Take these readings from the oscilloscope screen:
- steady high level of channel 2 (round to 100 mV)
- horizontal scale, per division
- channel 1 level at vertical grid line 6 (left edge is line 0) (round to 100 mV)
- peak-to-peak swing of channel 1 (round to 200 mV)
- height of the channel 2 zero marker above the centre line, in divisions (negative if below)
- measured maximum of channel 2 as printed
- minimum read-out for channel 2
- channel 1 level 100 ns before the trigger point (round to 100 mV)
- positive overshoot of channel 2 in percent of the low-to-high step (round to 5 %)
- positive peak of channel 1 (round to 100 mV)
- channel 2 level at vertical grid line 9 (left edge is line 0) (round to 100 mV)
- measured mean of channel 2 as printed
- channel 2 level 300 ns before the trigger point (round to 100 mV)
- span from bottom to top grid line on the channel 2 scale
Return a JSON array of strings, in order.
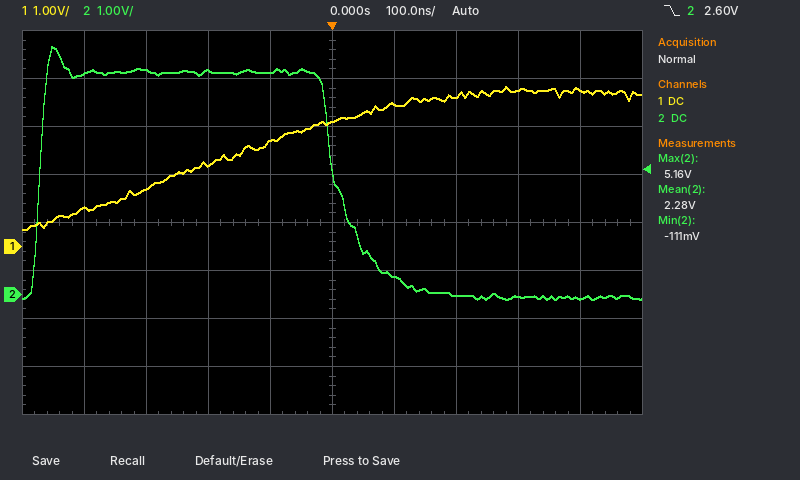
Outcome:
["4.6 V", "100 ns", "3.0 V", "3.0 V", "-1.5 div", "5.16 V", "-111 mV", "2.2 V", "10 %", "3.3 V", "-100 mV", "2.28 V", "4.7 V", "8 V"]
